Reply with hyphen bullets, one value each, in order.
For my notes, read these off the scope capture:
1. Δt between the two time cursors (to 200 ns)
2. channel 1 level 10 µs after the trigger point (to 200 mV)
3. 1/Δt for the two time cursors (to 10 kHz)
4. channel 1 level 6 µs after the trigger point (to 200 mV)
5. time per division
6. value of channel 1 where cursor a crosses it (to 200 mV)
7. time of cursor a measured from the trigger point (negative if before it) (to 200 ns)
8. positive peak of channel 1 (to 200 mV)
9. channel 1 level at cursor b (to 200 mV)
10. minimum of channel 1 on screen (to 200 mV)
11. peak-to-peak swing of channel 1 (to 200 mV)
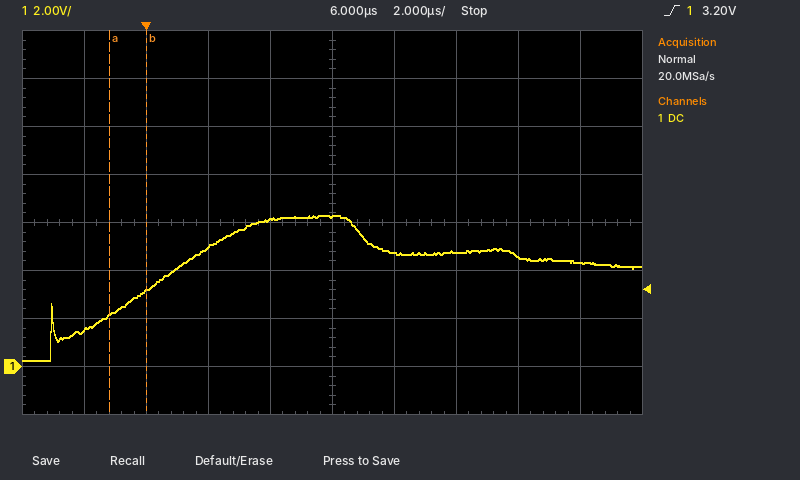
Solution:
- 1.2 µs
- 4.8 V
- 830 kHz
- 6.2 V
- 2 µs
- 2.2 V
- -1.2 µs
- 6.2 V
- 3.2 V
- 200 mV
- 6.0 V
